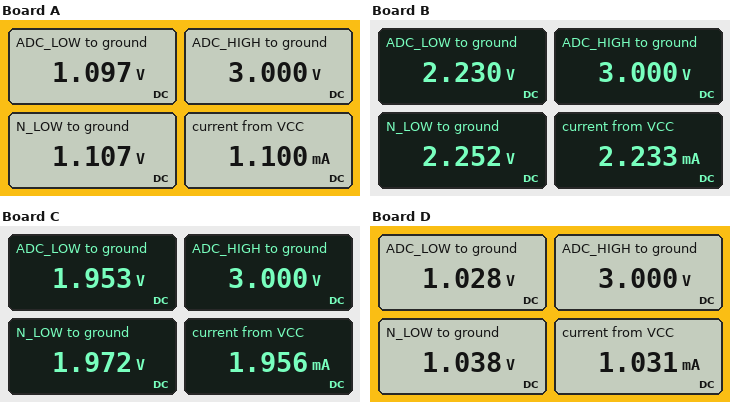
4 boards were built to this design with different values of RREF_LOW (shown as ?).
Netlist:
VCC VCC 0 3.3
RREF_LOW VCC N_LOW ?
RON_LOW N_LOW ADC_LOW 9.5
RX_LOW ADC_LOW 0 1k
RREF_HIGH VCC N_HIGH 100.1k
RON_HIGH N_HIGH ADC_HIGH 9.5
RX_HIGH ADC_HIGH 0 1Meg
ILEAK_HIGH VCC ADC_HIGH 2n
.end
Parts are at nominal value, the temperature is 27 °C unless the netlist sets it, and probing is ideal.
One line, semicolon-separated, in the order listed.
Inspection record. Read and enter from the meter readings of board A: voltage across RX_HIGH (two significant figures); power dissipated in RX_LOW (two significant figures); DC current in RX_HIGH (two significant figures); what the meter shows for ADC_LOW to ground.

3.0 V; 1.2 mW; 3.0 µA; 1.097 V
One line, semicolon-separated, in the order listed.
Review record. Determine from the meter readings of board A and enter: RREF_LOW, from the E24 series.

2 kΩ
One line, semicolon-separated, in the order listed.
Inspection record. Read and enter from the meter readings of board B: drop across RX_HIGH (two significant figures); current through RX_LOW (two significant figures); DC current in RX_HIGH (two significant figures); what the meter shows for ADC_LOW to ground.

3.0 V; 2.2 mA; 3.0 µA; 2.230 V
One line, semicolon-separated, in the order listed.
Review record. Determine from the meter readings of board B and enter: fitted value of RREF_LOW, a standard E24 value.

470 Ω
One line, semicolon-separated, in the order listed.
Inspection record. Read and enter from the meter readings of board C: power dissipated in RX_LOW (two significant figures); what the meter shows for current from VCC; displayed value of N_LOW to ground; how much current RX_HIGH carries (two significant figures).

3.8 mW; 1.956 mA; 1.972 V; 3.0 µA
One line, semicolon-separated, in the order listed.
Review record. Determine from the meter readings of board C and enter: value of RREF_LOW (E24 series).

680 Ω
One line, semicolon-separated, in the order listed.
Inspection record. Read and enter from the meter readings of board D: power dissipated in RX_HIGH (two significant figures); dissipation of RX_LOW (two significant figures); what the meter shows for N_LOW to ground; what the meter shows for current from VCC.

9.0 µW; 1.1 mW; 1.038 V; 1.031 mA
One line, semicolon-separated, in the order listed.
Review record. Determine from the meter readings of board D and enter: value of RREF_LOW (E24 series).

2.2 kΩ
